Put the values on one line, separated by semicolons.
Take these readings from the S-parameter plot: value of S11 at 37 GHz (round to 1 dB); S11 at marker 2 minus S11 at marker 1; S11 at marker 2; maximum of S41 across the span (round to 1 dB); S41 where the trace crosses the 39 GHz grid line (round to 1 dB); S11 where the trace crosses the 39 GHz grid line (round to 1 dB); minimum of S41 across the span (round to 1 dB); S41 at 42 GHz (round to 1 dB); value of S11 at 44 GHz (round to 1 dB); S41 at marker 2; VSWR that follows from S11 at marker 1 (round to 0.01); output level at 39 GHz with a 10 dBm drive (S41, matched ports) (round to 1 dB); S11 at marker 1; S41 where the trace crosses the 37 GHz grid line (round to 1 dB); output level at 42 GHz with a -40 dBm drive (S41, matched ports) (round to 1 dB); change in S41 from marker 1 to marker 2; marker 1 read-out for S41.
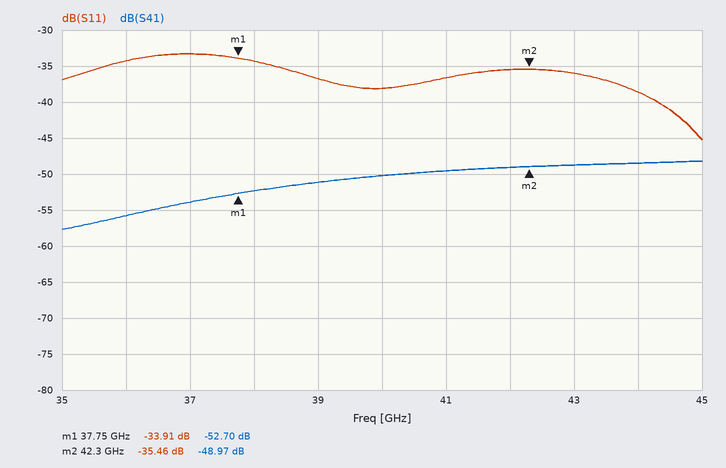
-33 dB; -1.55 dB; -35.46 dB; -48 dB; -51 dB; -37 dB; -58 dB; -49 dB; -39 dB; -48.97 dB; 1.04; -41 dBm; -33.91 dB; -54 dB; -89 dBm; 3.73 dB; -52.70 dB
